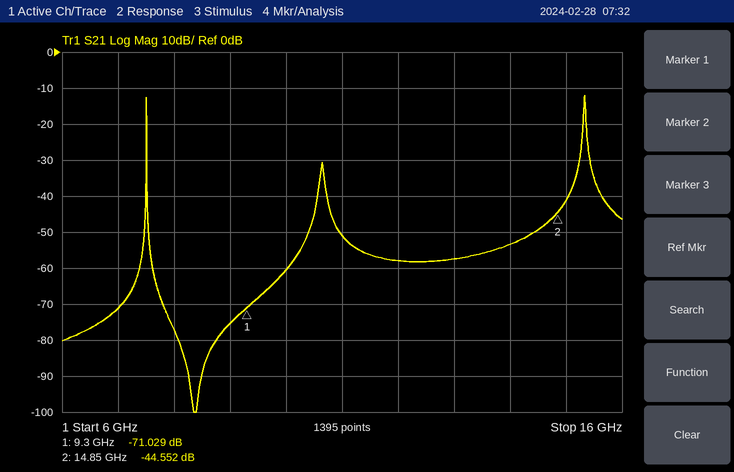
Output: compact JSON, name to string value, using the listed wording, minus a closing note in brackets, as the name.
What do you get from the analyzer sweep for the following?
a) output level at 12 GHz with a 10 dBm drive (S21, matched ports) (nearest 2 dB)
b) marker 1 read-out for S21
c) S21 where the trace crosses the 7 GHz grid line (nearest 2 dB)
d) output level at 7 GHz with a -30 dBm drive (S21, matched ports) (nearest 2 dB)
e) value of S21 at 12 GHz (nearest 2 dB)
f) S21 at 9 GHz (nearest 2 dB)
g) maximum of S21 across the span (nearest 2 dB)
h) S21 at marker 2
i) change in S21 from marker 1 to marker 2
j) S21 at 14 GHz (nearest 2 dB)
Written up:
{"output level at 12 GHz with a 10 dBm drive (S21, matched ports)": "-48 dBm", "marker 1 read-out for S21": "-71.029 dB", "S21 where the trace crosses the 7 GHz grid line": "-72 dB", "output level at 7 GHz with a -30 dBm drive (S21, matched ports)": "-102 dBm", "value of S21 at 12 GHz": "-58 dB", "S21 at 9 GHz": "-76 dB", "maximum of S21 across the span": "-12 dB", "S21 at marker 2": "-44.552 dB", "change in S21 from marker 1 to marker 2": "26.477 dB", "S21 at 14 GHz": "-54 dB"}
